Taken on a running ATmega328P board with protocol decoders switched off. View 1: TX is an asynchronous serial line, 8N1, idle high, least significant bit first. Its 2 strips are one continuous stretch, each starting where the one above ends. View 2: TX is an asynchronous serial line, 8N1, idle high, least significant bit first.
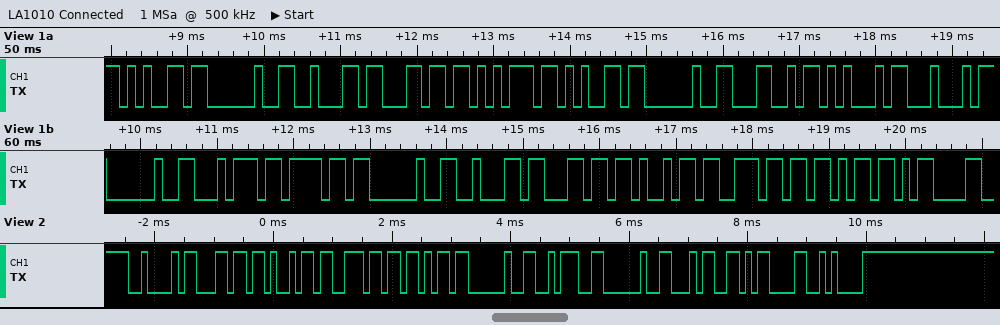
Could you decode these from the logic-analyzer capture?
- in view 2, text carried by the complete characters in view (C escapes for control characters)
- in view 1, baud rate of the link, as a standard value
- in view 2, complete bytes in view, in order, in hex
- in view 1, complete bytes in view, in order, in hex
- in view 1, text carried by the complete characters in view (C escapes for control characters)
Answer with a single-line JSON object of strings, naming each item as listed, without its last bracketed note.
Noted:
{"in view 2, text carried by the complete characters in view": "\"Blink : 4\\r\\n\"", "in view 1, baud rate of the link, as a standard value": "9600 baud", "in view 2, complete bytes in view, in order, in hex": "42 6C 69 6E 6B 20 3A 20 34 0D 0A", "in view 1, complete bytes in view, in order, in hex": "0x65 0x20 0x62 0x6C 0x75 0x65 0x20 0x4C 0x45 0x44 0x20 0x74 0x6F 0x20 0x62 0x6C 0x69 0x6E 0x6B 0x0D", "in view 1, text carried by the complete characters in view": "\"e blue LED to blink\\r\""}
